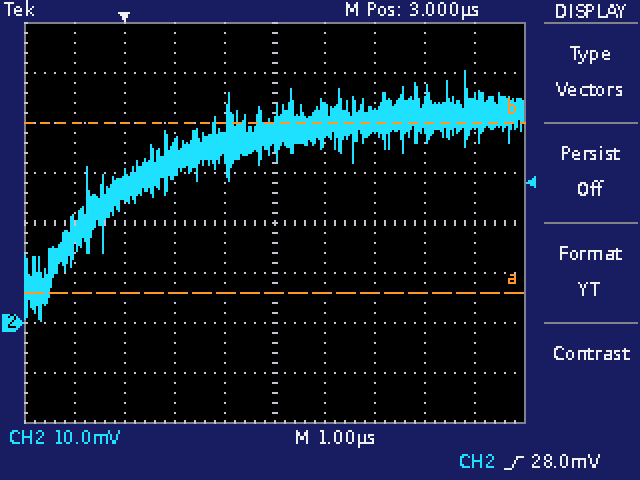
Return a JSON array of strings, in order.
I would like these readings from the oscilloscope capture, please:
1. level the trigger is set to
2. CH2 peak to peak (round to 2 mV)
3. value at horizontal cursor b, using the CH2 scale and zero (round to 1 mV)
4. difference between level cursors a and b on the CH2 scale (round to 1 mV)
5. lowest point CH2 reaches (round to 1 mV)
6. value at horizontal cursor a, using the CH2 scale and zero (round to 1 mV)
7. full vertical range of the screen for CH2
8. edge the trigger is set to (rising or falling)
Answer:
["28.0 mV", "50 mV", "40 mV", "34 mV", "0 mV", "6 mV", "80 mV", "rising"]
